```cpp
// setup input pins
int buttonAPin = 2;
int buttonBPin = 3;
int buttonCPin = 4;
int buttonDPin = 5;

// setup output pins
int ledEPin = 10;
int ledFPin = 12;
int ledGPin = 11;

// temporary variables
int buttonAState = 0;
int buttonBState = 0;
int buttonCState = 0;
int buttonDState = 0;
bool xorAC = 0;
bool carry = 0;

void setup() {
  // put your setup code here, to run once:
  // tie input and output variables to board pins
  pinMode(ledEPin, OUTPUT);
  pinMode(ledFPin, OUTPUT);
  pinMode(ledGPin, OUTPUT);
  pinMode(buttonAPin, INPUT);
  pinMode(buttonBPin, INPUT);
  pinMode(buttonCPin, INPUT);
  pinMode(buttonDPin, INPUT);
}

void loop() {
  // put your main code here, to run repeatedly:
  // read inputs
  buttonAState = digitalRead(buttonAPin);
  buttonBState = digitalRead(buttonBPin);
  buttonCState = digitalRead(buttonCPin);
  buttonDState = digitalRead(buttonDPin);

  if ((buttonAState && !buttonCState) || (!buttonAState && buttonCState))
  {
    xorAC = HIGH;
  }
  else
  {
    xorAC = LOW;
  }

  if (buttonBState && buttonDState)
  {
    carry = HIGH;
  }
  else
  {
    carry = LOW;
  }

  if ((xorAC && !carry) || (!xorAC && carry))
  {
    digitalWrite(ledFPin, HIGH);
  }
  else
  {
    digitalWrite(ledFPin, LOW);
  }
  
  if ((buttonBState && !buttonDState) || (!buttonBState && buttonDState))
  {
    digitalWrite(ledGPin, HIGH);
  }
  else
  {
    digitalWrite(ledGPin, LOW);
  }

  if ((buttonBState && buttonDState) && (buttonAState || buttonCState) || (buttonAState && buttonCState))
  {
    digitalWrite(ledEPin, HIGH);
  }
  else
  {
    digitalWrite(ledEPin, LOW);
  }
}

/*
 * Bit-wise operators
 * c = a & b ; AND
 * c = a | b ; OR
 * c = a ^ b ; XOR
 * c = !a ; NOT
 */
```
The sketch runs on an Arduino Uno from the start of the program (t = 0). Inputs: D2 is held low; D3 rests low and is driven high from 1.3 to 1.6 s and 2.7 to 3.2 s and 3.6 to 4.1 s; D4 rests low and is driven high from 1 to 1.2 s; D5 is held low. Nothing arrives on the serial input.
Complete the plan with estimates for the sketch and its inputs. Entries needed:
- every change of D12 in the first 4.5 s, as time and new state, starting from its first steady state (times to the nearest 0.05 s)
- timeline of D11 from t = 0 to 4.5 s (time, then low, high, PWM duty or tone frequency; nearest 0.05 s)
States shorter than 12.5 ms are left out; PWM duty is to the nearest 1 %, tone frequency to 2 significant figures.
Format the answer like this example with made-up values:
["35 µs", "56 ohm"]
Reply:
["0 s low; 1 s high; 1.2 s low", "0 s low; 1.3 s high; 1.6 s low; 2.7 s high; 3.2 s low; 3.6 s high; 4.1 s low"]
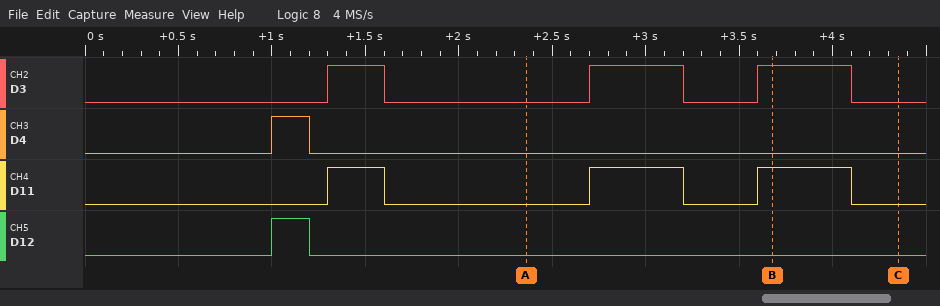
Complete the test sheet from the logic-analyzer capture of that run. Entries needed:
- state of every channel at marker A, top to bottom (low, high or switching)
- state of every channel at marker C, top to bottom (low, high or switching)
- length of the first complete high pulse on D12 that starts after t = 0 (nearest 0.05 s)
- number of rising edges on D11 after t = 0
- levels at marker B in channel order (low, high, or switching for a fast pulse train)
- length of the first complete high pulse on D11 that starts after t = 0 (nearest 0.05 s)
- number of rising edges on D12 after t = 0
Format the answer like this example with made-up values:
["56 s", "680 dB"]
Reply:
["D3 low, D4 low, D11 low, D12 low", "D3 low, D4 low, D11 low, D12 low", "0.20 s", "3", "D3 high, D4 low, D11 high, D12 low", "0.30 s", "1"]
